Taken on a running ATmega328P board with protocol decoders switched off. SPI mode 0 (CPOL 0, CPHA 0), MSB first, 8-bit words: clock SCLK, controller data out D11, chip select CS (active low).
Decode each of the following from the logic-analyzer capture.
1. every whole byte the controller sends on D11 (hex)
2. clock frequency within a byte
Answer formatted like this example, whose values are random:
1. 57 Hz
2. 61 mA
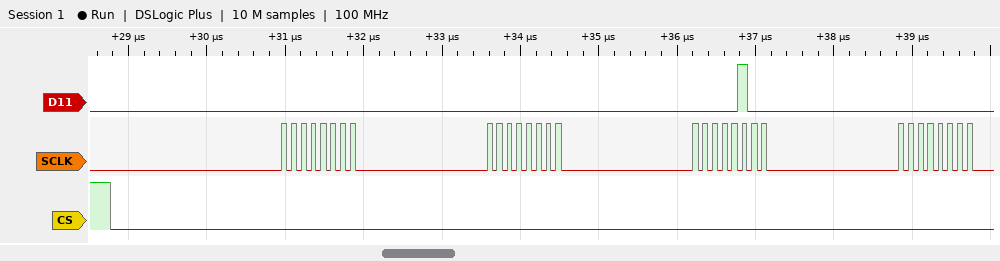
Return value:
1. 00 00 04 00
2. 8 MHz
